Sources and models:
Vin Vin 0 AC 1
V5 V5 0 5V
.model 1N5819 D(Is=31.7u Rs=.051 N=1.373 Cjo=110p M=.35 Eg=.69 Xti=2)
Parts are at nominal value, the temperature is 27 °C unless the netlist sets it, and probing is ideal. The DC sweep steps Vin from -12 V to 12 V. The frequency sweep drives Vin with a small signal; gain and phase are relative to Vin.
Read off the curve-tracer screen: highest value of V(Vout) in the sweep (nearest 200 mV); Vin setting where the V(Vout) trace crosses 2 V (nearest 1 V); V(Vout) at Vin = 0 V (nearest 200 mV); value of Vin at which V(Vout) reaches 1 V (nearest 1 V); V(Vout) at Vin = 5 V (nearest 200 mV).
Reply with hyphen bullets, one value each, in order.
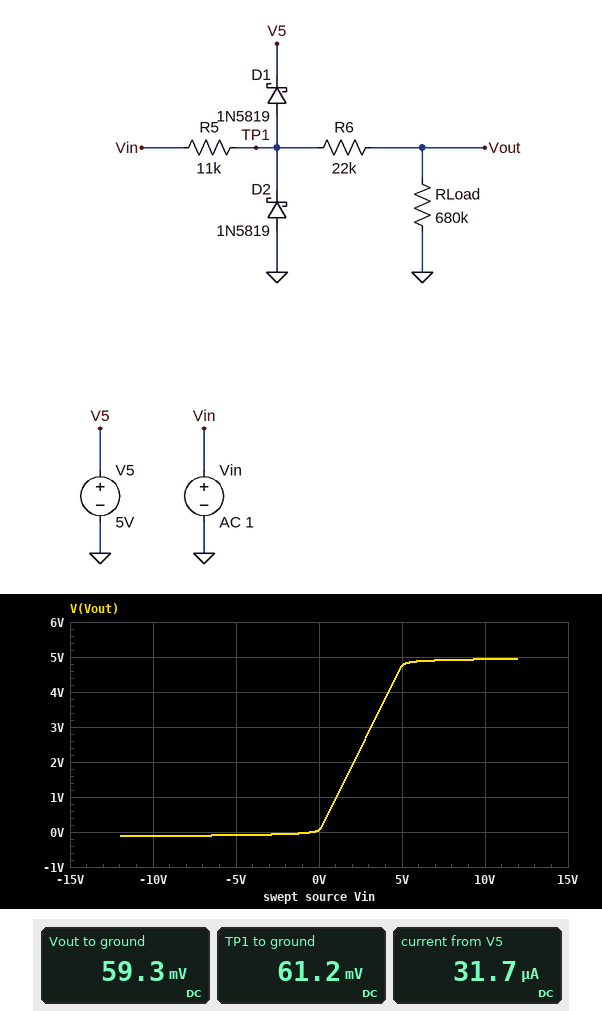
- 5.0 V
- 2 V
- 0 V
- 1 V
- 4.8 V
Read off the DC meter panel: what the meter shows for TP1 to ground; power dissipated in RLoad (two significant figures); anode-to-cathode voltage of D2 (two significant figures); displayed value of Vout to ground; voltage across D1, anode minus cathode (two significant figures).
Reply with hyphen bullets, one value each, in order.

- 61.2 mV
- 5.2 nW
- -61 mV
- 59.3 mV
- -4.9 V
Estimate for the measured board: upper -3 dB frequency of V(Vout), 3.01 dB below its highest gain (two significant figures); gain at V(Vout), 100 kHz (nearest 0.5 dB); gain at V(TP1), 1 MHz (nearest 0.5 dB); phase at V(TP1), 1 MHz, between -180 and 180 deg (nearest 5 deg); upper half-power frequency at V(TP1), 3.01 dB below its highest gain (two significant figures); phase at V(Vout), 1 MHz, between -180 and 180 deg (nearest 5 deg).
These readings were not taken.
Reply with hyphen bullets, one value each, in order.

- 240 kHz
- -10.0 dB
- -21.5 dB
- -75 deg
- 240 kHz
- -75 deg
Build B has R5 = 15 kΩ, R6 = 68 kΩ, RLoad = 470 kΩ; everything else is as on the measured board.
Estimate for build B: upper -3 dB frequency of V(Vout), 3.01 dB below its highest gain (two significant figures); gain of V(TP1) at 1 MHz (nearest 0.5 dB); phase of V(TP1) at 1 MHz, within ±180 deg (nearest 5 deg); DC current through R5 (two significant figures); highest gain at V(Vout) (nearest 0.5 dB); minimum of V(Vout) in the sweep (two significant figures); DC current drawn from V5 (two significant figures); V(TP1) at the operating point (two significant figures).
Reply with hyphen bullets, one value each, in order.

- 190 kHz
- -24.0 dB
- -80 deg
- 4.5 µA
- -10.5 dB
- -100 mV
- 32 µA
- 68 mV
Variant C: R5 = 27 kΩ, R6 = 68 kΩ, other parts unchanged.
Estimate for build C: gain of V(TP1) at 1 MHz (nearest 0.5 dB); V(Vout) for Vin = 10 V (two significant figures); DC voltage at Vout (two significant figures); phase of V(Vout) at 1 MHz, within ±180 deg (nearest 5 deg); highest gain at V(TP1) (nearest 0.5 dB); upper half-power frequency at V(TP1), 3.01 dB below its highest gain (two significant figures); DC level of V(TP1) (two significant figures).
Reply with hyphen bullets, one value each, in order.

- -29.0 dB
- 4.6 V
- 75 mV
- -85 deg
- -10.5 dB
- 120 kHz
- 82 mV
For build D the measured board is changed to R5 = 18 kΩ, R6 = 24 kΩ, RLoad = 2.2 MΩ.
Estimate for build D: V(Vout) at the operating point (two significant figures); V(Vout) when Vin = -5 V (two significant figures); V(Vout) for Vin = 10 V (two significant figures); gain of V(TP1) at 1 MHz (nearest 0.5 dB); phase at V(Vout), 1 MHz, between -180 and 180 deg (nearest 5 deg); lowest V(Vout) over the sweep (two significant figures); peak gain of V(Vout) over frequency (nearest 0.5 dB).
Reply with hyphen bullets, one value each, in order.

- 72 mV
- -76 mV
- 5.0 V
- -25.5 dB
- -80 deg
- -110 mV
- -10.0 dB
